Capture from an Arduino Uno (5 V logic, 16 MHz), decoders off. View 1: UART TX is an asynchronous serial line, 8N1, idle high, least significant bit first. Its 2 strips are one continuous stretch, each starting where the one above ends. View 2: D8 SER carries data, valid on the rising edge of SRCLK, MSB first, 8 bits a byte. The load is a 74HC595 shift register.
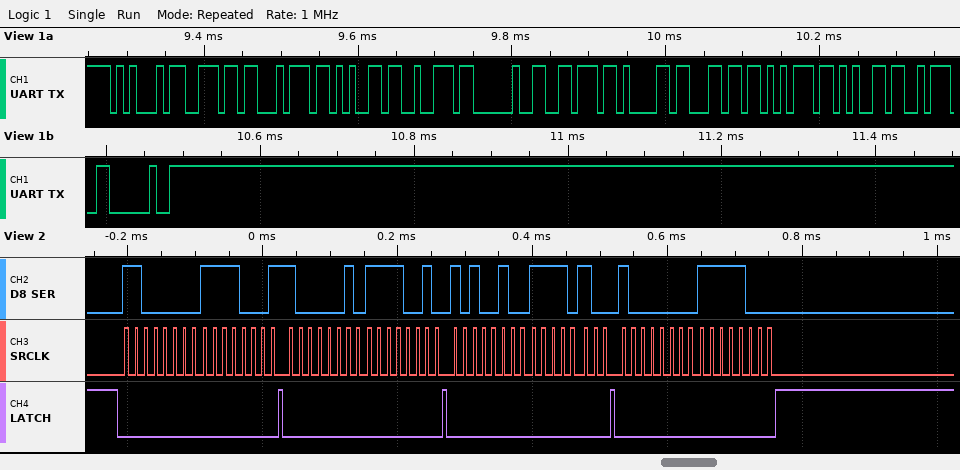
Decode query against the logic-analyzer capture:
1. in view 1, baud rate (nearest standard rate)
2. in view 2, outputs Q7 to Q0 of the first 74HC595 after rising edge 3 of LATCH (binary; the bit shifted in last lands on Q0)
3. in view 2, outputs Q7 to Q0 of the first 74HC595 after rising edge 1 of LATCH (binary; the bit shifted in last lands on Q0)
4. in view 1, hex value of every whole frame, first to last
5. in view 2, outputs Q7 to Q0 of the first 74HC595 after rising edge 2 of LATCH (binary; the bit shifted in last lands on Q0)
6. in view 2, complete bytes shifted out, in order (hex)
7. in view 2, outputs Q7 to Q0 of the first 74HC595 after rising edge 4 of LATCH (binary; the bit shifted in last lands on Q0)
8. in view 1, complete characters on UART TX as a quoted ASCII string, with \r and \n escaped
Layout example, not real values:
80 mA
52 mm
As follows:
115200 baud
11110100
11110001
45 6E 74 65 72 20 76 61 6C 75 65 3A 20
11110010
C0 F1 82 F2 A4 F4 80 F8
11111000
"Enter value: "
